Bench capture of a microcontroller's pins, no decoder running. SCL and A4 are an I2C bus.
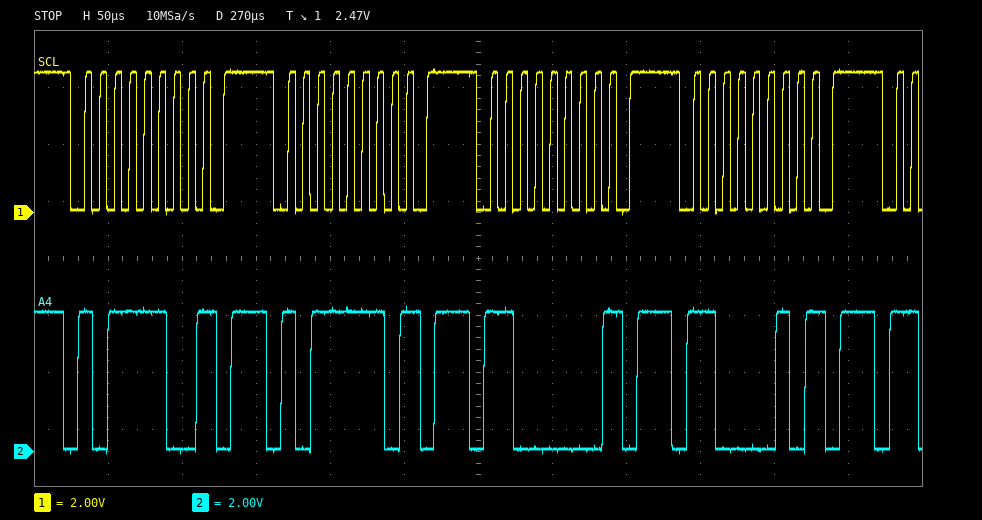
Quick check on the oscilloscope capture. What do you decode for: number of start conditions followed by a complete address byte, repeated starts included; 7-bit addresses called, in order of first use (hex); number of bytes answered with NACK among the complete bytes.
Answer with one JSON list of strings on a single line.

["4", "0x5E 0x5F 0x60 0x61", "4"]
